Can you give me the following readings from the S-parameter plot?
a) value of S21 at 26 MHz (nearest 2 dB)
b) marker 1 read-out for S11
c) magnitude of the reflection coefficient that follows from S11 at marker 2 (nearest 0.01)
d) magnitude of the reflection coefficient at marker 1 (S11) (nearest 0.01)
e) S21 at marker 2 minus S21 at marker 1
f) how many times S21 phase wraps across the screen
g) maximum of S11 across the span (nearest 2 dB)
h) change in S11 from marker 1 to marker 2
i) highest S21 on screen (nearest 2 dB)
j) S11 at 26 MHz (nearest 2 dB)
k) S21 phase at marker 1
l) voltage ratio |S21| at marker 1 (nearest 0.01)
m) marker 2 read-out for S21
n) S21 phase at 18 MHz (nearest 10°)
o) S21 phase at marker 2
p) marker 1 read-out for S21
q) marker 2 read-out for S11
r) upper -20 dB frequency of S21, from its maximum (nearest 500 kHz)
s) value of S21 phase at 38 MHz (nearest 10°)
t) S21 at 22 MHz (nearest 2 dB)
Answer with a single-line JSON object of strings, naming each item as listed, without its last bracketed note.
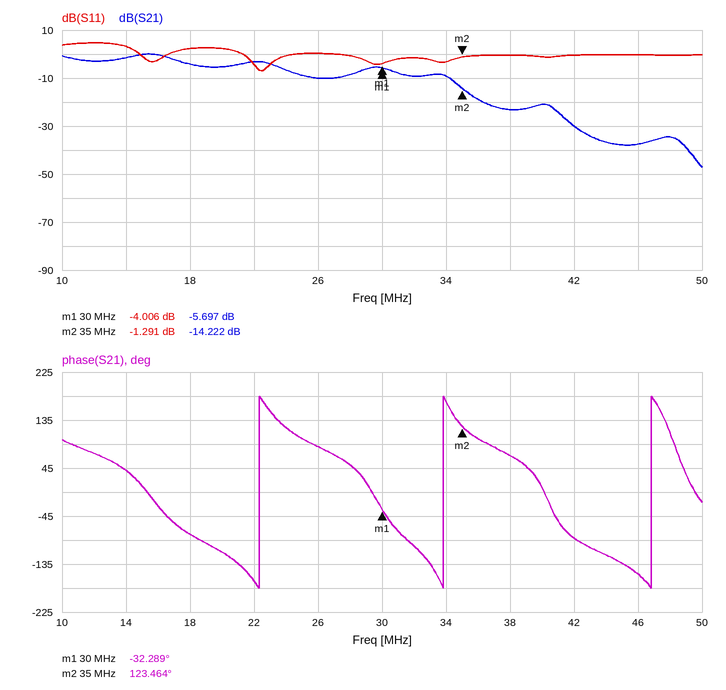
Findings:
{"value of S21 at 26 MHz": "-10 dB", "marker 1 read-out for S11": "-4.006 dB", "magnitude of the reflection coefficient that follows from S11 at marker 2": "0.86", "magnitude of the reflection coefficient at marker 1 (S11)": "0.63", "S21 at marker 2 minus S21 at marker 1": "-8.525 dB", "how many times S21 phase wraps across the screen": "3", "maximum of S11 across the span": "4 dB", "change in S11 from marker 1 to marker 2": "2.715 dB", "highest S21 on screen": "0 dB", "S11 at 26 MHz": "0 dB", "S21 phase at marker 1": "-32.289°", "voltage ratio |S21| at marker 1": "0.52", "marker 2 read-out for S21": "-14.222 dB", "S21 phase at 18 MHz": "-80°", "S21 phase at marker 2": "123.464°", "marker 1 read-out for S21": "-5.697 dB", "marker 2 read-out for S11": "-1.291 dB", "upper -20 dB frequency of S21, from its maximum": "36.5 MHz", "value of S21 phase at 38 MHz": "70°", "S21 at 22 MHz": "-4 dB"}
